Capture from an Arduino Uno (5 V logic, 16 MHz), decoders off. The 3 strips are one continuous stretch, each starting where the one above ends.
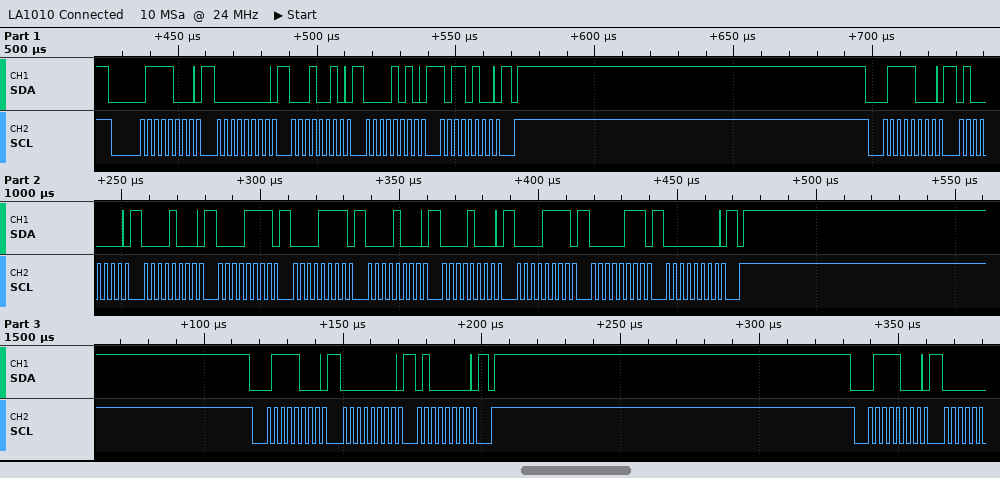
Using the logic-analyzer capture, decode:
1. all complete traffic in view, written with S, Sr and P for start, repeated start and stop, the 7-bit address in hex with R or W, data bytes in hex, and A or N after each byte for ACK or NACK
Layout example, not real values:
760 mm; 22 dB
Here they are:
S 3CW A 00 A 12 A 0A A B4 A P S 3CW A 40 A 08 A 0F A 0F A 08 A 08 A 0F A 07 A 00 A P S 3CW A 00 A 40 A P S 3CW A
